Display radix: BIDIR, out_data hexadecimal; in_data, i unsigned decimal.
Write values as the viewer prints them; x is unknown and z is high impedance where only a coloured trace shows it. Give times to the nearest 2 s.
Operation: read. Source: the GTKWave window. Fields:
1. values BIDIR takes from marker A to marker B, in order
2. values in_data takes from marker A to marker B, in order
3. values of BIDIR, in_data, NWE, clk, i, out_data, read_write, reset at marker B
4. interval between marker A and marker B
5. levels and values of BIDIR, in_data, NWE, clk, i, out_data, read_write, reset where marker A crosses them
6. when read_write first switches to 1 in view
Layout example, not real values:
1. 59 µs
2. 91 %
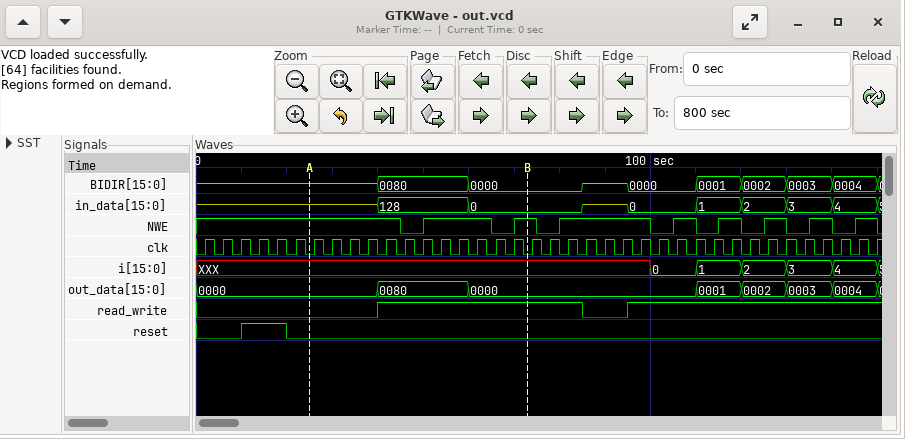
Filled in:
1. z, 0080, 0000
2. z, 128, 0
3. BIDIR=0000, in_data=0, NWE=1, clk=0, i=XXX, out_data=0000, read_write=1, reset=0
4. 48 s
5. BIDIR=z, in_data=z, NWE=1, clk=0, i=XXX, out_data=0000, read_write=0, reset=0
6. 40 s
